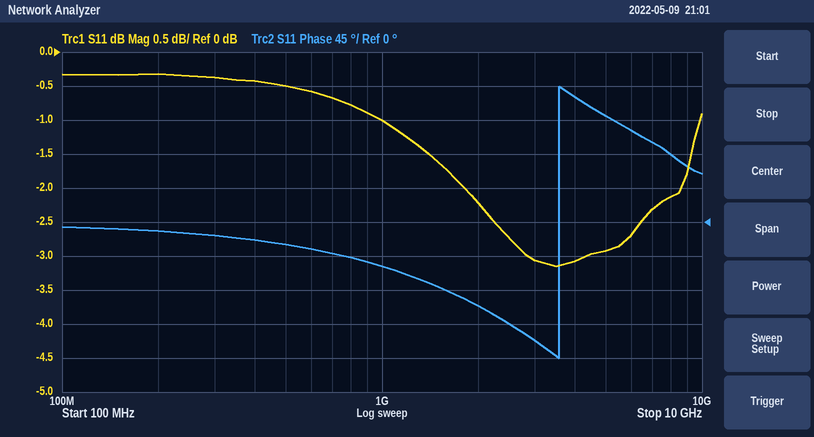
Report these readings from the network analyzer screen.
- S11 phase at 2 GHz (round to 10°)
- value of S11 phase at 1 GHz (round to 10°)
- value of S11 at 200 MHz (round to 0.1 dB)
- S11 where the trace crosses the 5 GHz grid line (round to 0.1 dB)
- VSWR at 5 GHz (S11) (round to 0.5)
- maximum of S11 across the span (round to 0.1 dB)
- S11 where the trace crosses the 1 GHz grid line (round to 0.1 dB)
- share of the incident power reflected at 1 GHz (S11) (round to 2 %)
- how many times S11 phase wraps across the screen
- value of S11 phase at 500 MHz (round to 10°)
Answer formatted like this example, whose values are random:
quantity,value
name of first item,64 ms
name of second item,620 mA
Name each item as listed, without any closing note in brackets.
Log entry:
quantity,value
S11 phase at 2 GHz,-110°
value of S11 phase at 1 GHz,-60°
value of S11 at 200 MHz,-0.3 dB
S11 where the trace crosses the 5 GHz grid line,-2.9 dB
VSWR at 5 GHz (S11),6.0
maximum of S11 across the span,-0.3 dB
S11 where the trace crosses the 1 GHz grid line,-1.0 dB
share of the incident power reflected at 1 GHz (S11),80 %
how many times S11 phase wraps across the screen,1
value of S11 phase at 500 MHz,-30°
